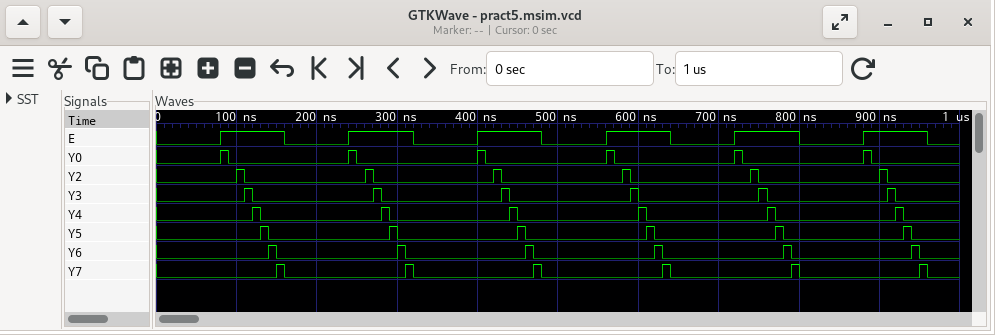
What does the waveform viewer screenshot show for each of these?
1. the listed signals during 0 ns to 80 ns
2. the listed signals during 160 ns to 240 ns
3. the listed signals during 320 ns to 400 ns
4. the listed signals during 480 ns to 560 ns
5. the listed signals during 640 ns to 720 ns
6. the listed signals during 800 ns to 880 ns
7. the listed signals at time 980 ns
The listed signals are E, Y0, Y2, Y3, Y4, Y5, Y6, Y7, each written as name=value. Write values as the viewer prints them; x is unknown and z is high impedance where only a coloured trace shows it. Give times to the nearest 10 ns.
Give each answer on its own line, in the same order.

E=0, Y0=0, Y2=0, Y3=0, Y4=0, Y5=0, Y6=0, Y7=0
E=0, Y0=0, Y2=0, Y3=0, Y4=0, Y5=0, Y6=0, Y7=0
E=0, Y0=0, Y2=0, Y3=0, Y4=0, Y5=0, Y6=0, Y7=0
E=0, Y0=0, Y2=0, Y3=0, Y4=0, Y5=0, Y6=0, Y7=0
E=0, Y0=0, Y2=0, Y3=0, Y4=0, Y5=0, Y6=0, Y7=0
E=0, Y0=0, Y2=0, Y3=0, Y4=0, Y5=0, Y6=0, Y7=0
E=0, Y0=0, Y2=0, Y3=0, Y4=0, Y5=0, Y6=0, Y7=0
